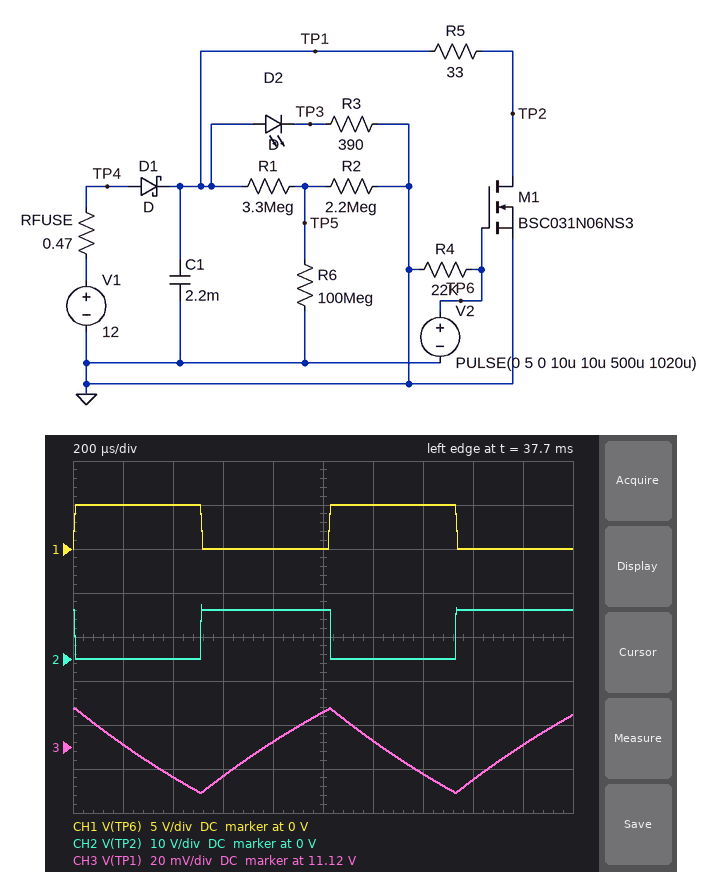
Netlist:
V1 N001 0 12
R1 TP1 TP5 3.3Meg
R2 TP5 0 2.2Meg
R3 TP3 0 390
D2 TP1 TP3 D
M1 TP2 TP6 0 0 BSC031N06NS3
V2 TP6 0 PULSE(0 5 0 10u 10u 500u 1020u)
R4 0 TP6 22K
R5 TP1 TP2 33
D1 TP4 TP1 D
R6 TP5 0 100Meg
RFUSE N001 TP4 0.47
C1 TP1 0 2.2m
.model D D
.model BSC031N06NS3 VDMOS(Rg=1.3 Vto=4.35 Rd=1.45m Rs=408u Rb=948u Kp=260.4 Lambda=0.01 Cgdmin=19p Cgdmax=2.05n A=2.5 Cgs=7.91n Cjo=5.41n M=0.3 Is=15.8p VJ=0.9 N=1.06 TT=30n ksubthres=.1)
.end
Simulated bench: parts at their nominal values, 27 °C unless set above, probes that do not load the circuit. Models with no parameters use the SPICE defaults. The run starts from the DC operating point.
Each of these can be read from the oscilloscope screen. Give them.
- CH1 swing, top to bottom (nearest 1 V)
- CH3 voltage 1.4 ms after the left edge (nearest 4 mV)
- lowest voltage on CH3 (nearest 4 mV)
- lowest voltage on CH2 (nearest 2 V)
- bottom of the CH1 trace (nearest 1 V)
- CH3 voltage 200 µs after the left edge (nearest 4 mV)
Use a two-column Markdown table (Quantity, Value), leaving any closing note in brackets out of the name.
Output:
| Quantity | Value |
|---|---|
| CH1 swing, top to bottom | 5 V |
| CH3 voltage 1.4 ms after the left edge | 11.108 V |
| lowest voltage on CH3 | 11.100 V |
| lowest voltage on CH2 | 0 V |
| bottom of the CH1 trace | 0 V |
| CH3 voltage 200 µs after the left edge | 11.120 V |
